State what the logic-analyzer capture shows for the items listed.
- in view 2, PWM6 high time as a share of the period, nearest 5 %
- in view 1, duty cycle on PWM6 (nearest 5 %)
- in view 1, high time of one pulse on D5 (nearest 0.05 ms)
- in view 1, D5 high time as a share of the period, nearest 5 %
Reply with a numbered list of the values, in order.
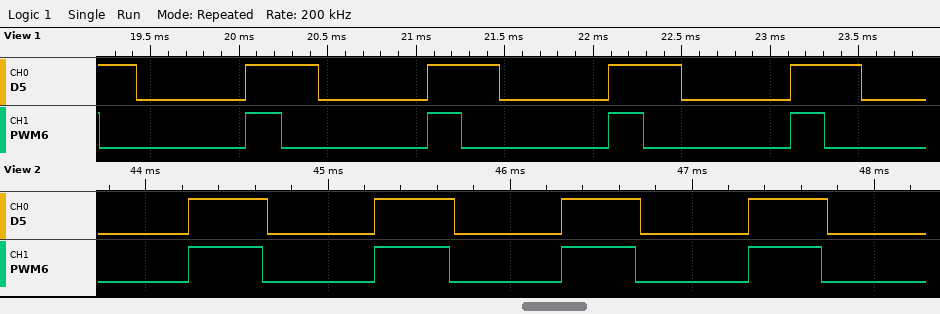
1. 40 %
2. 20 %
3. 0.40 ms
4. 40 %
